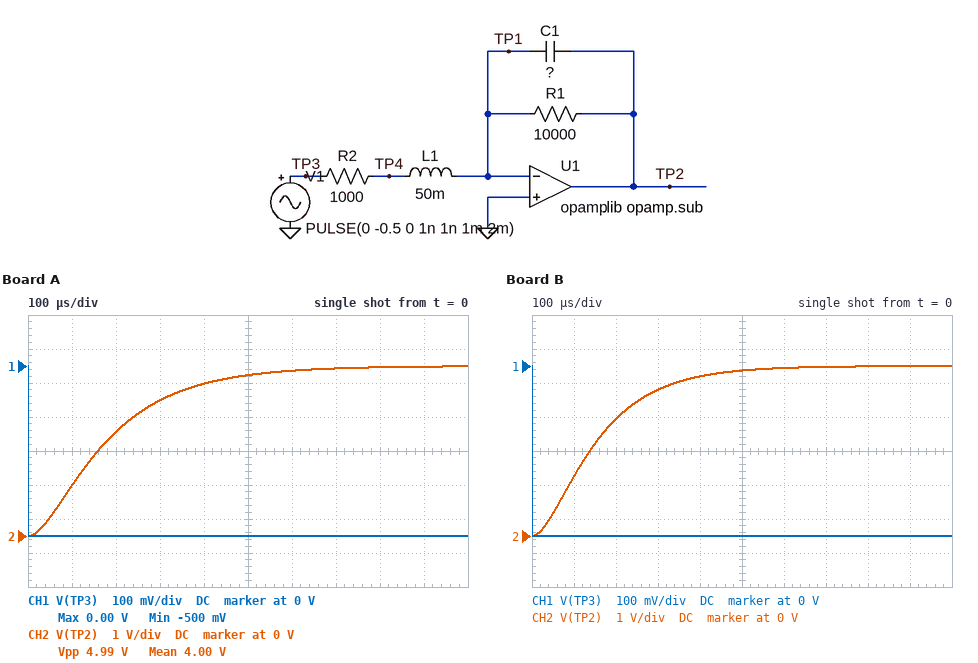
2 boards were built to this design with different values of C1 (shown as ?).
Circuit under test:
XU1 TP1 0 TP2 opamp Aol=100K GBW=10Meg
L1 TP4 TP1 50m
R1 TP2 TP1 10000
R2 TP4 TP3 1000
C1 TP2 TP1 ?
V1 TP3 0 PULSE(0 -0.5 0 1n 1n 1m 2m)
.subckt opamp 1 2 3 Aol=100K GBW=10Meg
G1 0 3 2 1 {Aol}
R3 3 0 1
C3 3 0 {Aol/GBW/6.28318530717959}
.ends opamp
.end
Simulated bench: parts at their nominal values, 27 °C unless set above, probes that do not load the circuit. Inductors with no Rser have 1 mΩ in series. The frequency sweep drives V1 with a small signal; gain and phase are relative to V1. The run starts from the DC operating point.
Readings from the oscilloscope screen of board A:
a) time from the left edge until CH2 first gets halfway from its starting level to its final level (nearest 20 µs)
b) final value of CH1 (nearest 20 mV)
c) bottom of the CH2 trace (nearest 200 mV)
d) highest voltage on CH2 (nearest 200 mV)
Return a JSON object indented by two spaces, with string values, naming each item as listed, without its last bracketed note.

{
  "time from the left edge until CH2 first gets halfway from its starting level to its final level": "160 µs",
  "final value of CH1": "-500 mV",
  "bottom of the CH2 trace": "0 V",
  "highest voltage on CH2": "5.0 V"
}
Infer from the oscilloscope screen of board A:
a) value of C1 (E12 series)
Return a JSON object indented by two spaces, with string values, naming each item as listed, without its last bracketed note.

{
  "value of C1": "15 nF"
}
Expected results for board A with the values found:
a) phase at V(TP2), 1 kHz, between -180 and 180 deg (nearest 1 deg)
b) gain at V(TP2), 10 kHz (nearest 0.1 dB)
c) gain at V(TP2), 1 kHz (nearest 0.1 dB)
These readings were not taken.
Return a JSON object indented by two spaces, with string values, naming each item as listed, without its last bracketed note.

{
  "phase at V(TP2), 1 kHz, between -180 and 180 deg": "119 deg",
  "gain at V(TP2), 10 kHz": "-9.9 dB",
  "gain at V(TP2), 1 kHz": "16.8 dB"
}
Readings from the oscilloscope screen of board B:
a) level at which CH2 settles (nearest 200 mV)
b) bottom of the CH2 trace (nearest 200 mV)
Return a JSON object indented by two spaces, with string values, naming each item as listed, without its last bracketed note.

{
  "level at which CH2 settles": "5.0 V",
  "bottom of the CH2 trace": "0 V"
}
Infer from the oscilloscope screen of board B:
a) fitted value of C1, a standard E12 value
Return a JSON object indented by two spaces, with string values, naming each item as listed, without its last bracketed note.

{
  "fitted value of C1, a standard E12 value": "12 nF"
}
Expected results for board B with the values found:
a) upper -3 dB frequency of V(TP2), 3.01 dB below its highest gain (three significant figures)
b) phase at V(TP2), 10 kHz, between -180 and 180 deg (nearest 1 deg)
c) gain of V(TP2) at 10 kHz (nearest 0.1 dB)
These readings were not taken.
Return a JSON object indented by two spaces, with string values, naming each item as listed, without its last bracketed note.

{
  "upper -3 dB frequency of V(TP2), 3.01 dB below its highest gain": "1.16 kHz",
  "phase at V(TP2), 10 kHz, between -180 and 180 deg": "25 deg",
  "gain of V(TP2) at 10 kHz": "-8.0 dB"
}
